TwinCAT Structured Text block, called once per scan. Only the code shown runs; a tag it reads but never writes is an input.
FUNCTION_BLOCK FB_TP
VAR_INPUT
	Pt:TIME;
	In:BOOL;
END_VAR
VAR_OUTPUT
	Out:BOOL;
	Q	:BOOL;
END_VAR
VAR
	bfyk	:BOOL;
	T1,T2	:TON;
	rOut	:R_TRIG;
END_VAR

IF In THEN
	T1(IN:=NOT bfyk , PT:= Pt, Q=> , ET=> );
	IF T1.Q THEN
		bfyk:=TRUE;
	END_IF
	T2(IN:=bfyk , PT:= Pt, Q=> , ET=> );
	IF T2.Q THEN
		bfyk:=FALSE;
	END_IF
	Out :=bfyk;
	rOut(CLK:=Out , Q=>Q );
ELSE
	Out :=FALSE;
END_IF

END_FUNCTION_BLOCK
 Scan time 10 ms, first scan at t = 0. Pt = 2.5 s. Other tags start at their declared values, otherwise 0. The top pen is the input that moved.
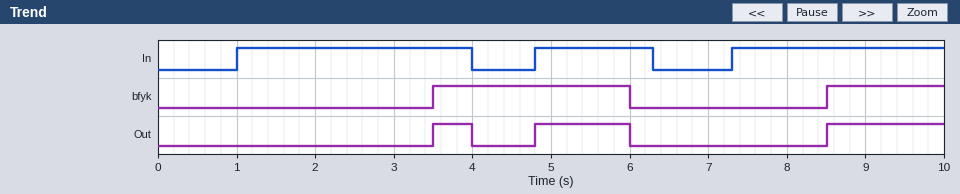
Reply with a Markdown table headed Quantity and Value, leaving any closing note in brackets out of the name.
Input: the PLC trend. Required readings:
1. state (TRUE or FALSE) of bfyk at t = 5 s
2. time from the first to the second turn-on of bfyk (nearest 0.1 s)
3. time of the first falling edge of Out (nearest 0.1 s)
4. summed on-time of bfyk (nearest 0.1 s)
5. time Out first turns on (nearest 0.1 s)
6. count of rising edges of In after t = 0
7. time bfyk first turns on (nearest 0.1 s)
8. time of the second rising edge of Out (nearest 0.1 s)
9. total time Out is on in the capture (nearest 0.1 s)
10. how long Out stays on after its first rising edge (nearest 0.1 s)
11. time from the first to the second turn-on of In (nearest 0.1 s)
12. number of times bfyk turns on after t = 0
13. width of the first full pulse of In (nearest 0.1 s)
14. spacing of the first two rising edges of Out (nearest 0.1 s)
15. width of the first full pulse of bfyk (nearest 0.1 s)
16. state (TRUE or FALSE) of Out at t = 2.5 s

| Quantity | Value |
|---|---|
| state (TRUE or FALSE) of bfyk at t = 5 s | TRUE |
| time from the first to the second turn-on of bfyk | 5.0 s |
| time of the first falling edge of Out | 4.0 s |
| summed on-time of bfyk | 4.0 s |
| time Out first turns on | 3.5 s |
| count of rising edges of In after t = 0 | 3 |
| time bfyk first turns on | 3.5 s |
| time of the second rising edge of Out | 4.8 s |
| total time Out is on in the capture | 3.2 s |
| how long Out stays on after its first rising edge | 0.5 s |
| time from the first to the second turn-on of In | 3.8 s |
| number of times bfyk turns on after t = 0 | 2 |
| width of the first full pulse of In | 3.0 s |
| spacing of the first two rising edges of Out | 1.3 s |
| width of the first full pulse of bfyk | 2.5 s |
| state (TRUE or FALSE) of Out at t = 2.5 s | FALSE |
